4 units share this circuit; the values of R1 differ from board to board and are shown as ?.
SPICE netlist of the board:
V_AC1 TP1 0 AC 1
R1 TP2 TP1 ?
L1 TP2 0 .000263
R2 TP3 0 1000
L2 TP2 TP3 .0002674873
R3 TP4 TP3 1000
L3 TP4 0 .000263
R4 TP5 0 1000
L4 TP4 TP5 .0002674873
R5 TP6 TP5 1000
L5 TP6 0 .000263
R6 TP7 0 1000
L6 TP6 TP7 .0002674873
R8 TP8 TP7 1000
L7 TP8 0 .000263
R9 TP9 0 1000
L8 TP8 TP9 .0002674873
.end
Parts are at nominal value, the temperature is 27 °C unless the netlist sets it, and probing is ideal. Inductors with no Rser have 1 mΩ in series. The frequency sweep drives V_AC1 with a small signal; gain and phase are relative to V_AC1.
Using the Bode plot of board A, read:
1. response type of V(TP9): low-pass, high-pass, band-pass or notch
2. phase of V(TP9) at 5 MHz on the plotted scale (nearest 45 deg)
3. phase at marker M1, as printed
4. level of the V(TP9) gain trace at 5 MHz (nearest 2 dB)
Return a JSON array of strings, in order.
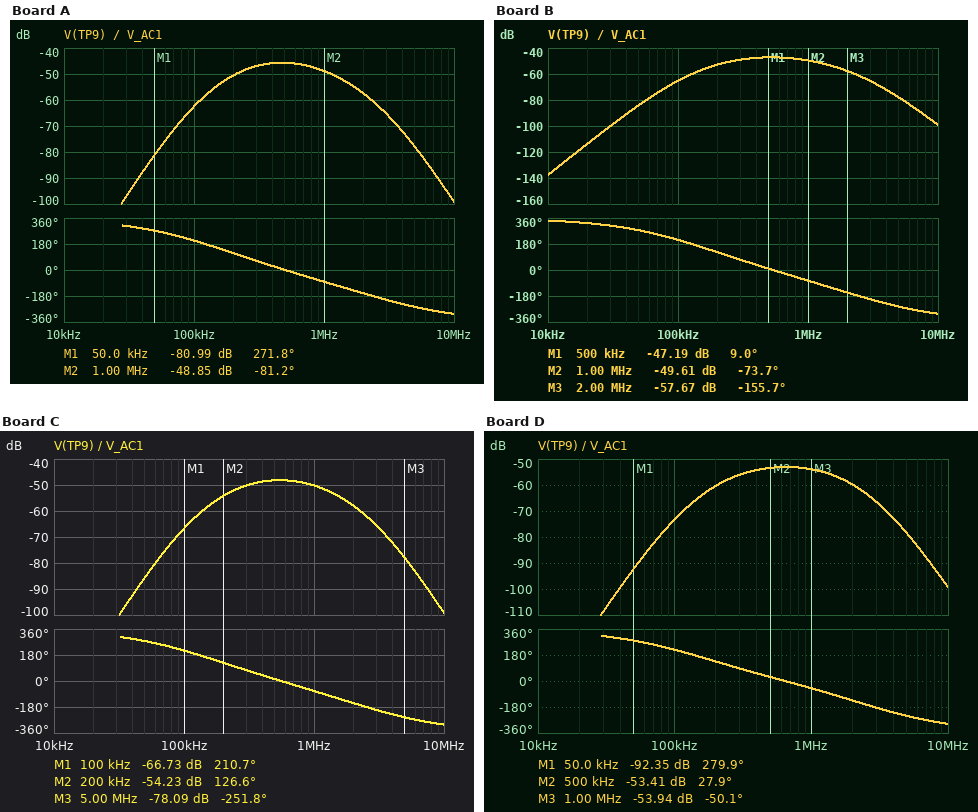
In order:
["band-pass", "-270 deg", "271.8 deg", "-78 dB"]
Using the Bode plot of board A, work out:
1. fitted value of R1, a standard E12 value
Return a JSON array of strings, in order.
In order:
["390 Ω"]
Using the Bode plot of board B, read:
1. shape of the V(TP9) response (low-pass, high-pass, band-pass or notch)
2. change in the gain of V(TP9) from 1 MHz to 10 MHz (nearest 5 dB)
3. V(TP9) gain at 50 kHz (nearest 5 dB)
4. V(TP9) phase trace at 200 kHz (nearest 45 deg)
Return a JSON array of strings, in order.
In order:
["band-pass", "-50 dB", "-85 dB", "135 deg"]
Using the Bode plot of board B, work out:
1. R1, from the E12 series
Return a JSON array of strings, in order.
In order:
["560 Ω"]
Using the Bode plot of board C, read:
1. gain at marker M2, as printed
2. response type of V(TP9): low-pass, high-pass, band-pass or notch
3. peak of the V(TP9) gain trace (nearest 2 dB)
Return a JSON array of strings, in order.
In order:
["-54.23 dB", "band-pass", "-48 dB"]
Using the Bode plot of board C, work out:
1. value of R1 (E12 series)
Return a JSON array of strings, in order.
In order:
["680 Ω"]
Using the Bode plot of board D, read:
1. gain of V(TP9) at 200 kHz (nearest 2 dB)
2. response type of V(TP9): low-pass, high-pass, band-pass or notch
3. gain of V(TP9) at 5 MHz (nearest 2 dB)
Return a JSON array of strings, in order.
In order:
["-60 dB", "band-pass", "-78 dB"]
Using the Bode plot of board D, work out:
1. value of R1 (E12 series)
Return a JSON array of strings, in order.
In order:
["1.5 kΩ"]
